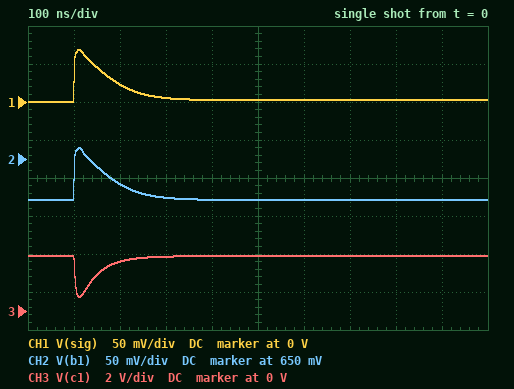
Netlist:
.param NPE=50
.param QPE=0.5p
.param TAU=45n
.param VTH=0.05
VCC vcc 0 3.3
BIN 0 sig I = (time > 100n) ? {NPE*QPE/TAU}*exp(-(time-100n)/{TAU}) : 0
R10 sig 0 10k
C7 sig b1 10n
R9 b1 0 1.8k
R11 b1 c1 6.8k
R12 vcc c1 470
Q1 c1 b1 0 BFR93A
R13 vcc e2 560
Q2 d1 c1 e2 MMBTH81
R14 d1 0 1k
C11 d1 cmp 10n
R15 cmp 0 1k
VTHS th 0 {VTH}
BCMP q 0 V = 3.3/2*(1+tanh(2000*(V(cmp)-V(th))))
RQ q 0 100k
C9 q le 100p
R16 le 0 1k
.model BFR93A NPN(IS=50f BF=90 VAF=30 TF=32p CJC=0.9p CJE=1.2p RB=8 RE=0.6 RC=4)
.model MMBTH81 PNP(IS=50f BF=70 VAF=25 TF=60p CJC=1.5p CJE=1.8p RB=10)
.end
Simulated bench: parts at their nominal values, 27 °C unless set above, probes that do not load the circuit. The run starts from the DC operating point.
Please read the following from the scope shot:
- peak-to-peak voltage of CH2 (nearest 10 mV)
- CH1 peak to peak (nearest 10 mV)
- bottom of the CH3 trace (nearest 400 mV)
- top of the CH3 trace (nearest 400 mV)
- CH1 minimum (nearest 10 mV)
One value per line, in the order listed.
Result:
70 mV
70 mV
800 mV
2.8 V
0 V
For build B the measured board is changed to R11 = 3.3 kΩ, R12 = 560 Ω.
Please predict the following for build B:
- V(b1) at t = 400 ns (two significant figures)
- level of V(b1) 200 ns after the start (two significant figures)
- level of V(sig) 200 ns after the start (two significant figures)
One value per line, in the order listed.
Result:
630 mV
640 mV
6.6 mV
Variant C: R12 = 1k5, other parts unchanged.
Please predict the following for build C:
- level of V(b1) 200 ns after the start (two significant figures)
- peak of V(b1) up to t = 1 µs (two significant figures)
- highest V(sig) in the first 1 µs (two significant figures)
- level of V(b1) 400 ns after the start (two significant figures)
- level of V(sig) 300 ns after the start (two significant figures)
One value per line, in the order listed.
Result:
580 mV
650 mV
93 mV
560 mV
6.3 mV
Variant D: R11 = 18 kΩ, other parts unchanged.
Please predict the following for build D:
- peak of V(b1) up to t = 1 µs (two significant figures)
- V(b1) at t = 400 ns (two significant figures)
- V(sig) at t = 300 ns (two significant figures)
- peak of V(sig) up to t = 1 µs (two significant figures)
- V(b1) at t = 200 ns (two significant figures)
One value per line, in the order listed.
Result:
650 mV
290 mV
12 mV
360 mV
380 mV
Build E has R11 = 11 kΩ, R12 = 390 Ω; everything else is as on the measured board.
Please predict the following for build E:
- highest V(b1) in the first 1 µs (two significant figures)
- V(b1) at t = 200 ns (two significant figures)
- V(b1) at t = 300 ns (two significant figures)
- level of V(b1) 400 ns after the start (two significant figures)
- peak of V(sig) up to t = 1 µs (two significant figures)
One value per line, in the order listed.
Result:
660 mV
530 mV
460 mV
450 mV
210 mV
